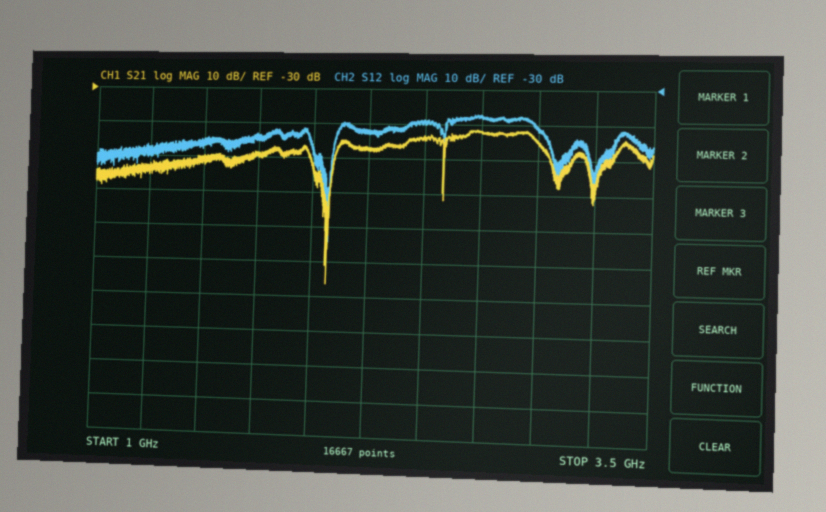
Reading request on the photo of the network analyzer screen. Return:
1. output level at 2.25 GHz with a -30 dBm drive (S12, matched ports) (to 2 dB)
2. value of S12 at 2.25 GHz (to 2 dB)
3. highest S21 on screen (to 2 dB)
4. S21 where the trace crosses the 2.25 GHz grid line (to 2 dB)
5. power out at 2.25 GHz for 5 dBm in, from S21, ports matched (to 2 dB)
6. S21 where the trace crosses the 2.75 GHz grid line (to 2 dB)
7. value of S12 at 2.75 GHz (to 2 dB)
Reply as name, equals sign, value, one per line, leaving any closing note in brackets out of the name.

output level at 2.25 GHz with a -30 dBm drive (S12, matched ports) = -72 dBm
value of S12 at 2.25 GHz = -42 dB
highest S21 on screen = -42 dB
S21 where the trace crosses the 2.25 GHz grid line = -48 dB
power out at 2.25 GHz for 5 dBm in, from S21, ports matched = -42 dBm
S21 where the trace crosses the 2.75 GHz grid line = -42 dB
value of S12 at 2.75 GHz = -38 dB
